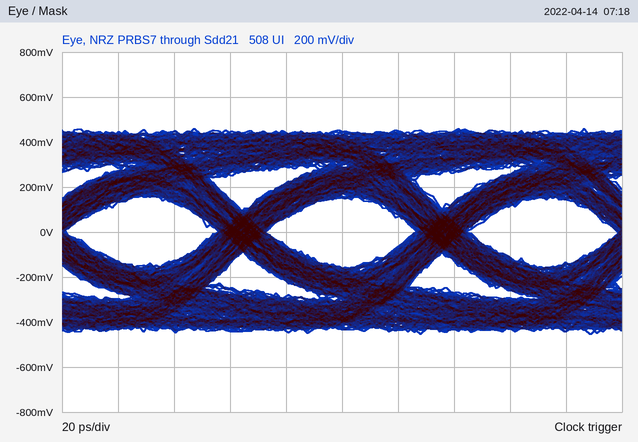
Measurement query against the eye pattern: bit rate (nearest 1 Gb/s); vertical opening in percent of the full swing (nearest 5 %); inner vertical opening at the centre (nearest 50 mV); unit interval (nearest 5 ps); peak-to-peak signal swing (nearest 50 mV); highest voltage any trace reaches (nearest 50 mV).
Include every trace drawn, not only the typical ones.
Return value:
14 Gb/s
35 %
300 mV
70 ps
900 mV
450 mV
